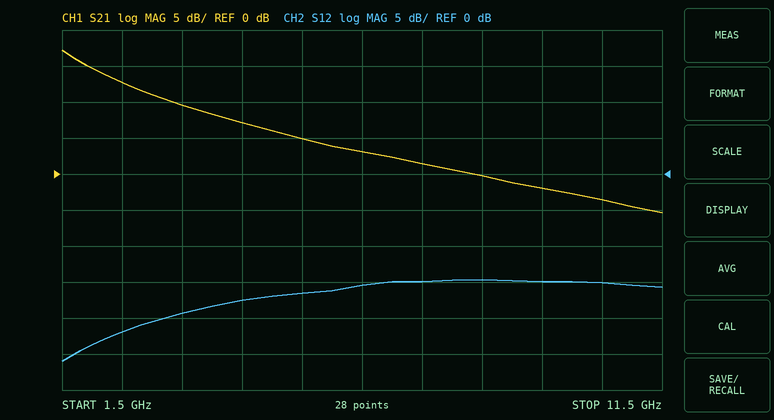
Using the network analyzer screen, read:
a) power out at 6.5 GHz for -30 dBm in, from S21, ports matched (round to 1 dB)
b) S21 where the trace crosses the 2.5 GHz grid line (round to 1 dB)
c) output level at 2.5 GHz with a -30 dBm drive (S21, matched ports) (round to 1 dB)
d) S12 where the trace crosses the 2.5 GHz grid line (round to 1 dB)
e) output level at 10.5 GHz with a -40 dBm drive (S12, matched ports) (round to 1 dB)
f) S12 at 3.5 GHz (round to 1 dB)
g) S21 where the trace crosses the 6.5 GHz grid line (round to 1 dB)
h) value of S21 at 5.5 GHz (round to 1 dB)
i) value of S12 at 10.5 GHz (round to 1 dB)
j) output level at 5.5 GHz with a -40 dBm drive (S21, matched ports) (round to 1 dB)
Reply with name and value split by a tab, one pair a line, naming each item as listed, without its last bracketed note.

power out at 6.5 GHz for -30 dBm in, from S21, ports matched	-27 dBm
S21 where the trace crosses the 2.5 GHz grid line	13 dB
output level at 2.5 GHz with a -30 dBm drive (S21, matched ports)	-17 dBm
S12 where the trace crosses the 2.5 GHz grid line	-22 dB
output level at 10.5 GHz with a -40 dBm drive (S12, matched ports)	-55 dBm
S12 at 3.5 GHz	-19 dB
S21 where the trace crosses the 6.5 GHz grid line	3 dB
value of S21 at 5.5 GHz	5 dB
value of S12 at 10.5 GHz	-15 dB
output level at 5.5 GHz with a -40 dBm drive (S21, matched ports)	-35 dBm
